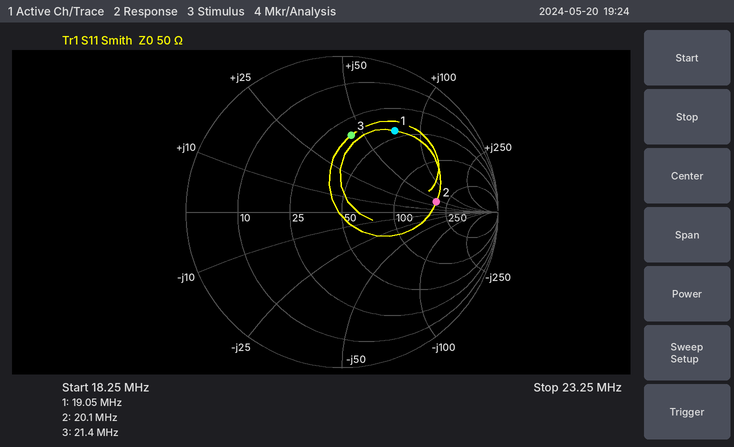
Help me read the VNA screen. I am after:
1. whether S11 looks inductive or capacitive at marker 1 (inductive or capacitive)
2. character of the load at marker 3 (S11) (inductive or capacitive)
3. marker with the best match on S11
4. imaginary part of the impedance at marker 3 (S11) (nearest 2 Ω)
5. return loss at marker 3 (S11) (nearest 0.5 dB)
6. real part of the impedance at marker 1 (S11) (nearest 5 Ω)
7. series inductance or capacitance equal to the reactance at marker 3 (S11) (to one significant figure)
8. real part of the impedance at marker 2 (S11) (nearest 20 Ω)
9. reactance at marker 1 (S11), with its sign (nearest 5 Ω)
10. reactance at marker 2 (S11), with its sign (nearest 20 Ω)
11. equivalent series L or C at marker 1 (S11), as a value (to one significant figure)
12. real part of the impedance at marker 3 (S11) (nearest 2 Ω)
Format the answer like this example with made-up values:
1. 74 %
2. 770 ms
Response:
1. inductive
2. inductive
3. marker 3
4. +44 Ω
5. 6.0 dB
6. 45 Ω
7. 300 nH
8. 200 Ω
9. +75 Ω
10. +40 Ω
11. 600 nH
12. 34 Ω
